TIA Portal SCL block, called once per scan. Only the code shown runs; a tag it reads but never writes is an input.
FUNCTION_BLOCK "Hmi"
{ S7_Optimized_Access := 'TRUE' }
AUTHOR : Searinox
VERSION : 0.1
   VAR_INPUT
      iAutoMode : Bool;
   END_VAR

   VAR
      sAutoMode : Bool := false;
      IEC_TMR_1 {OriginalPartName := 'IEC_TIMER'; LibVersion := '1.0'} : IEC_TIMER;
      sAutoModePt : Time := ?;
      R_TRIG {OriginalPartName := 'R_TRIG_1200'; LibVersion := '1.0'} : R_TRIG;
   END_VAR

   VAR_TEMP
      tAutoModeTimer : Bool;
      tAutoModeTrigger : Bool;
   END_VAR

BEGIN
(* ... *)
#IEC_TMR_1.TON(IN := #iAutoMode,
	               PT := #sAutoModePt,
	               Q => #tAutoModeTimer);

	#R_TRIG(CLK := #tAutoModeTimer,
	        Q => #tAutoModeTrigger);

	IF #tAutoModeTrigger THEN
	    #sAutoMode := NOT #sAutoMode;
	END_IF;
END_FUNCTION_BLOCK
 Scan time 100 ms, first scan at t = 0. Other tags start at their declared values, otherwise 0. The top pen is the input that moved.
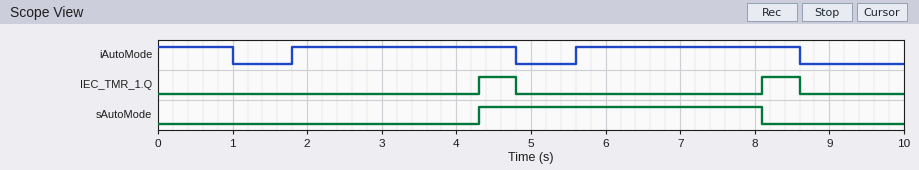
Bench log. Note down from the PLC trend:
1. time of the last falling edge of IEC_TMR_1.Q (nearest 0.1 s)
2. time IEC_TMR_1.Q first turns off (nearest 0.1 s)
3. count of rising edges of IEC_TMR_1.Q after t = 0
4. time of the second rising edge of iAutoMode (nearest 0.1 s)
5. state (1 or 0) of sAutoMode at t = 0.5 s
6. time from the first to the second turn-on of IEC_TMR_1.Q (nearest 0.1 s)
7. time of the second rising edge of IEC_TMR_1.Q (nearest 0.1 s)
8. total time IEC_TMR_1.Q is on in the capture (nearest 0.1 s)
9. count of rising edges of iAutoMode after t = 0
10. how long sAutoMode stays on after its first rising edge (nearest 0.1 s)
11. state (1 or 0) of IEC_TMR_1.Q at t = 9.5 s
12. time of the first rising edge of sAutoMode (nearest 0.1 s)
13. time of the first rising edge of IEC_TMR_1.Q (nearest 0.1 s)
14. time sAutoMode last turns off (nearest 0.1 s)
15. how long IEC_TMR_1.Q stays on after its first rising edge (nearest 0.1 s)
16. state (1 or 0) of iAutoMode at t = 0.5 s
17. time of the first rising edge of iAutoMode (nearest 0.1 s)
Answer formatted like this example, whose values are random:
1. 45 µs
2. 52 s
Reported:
1. 8.6 s
2. 4.8 s
3. 2
4. 5.6 s
5. 0
6. 3.8 s
7. 8.1 s
8. 1.0 s
9. 2
10. 3.8 s
11. 0
12. 4.3 s
13. 4.3 s
14. 8.1 s
15. 0.5 s
16. 1
17. 1.8 s
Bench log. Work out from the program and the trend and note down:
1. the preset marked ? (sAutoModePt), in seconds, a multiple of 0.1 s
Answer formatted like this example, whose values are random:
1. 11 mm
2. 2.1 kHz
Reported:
1. 2.5 s
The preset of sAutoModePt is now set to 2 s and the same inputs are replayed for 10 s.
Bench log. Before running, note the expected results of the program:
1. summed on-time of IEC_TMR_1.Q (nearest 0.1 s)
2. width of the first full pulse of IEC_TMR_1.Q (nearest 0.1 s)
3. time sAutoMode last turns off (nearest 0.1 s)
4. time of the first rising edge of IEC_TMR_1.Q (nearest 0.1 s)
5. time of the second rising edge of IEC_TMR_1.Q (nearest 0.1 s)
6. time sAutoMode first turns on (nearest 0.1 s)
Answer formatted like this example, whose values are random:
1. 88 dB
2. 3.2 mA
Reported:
1. 2.0 s
2. 1.0 s
3. 7.6 s
4. 3.8 s
5. 7.6 s
6. 3.8 s
